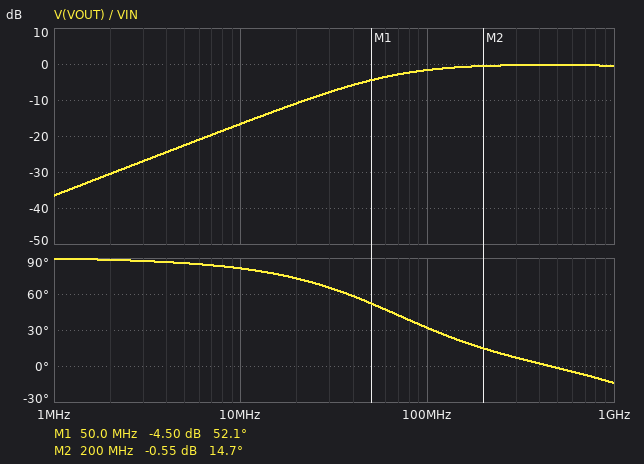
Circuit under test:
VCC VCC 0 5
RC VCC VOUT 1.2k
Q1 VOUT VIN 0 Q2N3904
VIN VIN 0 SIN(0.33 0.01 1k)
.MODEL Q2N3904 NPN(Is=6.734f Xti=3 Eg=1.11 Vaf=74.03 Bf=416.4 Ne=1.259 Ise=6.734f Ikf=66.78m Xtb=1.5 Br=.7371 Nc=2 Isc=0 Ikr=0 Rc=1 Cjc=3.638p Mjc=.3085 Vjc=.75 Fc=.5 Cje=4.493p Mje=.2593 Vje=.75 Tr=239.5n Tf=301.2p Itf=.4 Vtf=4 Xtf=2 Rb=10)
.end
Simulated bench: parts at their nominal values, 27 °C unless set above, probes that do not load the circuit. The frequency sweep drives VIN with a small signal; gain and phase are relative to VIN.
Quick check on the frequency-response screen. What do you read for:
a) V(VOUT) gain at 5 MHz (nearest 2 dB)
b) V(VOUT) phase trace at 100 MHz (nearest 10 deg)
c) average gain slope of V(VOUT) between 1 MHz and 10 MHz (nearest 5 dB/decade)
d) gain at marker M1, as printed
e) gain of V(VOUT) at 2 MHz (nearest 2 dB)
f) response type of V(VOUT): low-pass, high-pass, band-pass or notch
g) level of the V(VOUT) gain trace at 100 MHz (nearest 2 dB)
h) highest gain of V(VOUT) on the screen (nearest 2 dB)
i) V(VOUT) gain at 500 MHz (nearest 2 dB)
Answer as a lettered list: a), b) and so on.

a) -22 dB
b) 30 deg
c) 20 dB/decade
d) -4.50 dB
e) -30 dB
f) high-pass
g) -2 dB
h) 0 dB
i) 0 dB
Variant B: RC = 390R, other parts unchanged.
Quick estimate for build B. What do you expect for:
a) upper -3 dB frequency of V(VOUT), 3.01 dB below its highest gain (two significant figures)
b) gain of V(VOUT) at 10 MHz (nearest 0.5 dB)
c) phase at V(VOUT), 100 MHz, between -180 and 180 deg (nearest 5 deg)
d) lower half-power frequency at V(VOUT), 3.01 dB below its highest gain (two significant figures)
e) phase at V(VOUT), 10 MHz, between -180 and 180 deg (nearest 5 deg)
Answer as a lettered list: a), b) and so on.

a) 3.5 GHz
b) -26.5 dB
c) 60 deg
d) 180 MHz
e) 85 deg
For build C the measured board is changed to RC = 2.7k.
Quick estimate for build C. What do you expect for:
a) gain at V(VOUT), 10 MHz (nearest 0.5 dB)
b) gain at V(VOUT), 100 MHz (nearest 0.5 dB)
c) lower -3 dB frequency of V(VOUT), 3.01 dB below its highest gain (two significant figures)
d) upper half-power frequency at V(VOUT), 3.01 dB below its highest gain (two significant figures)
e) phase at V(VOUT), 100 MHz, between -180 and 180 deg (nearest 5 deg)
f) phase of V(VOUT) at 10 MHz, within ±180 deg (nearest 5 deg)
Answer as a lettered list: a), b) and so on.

a) -10.0 dB
b) -0.5 dB
c) 29 MHz
d) 3.1 GHz
e) 15 deg
f) 70 deg
